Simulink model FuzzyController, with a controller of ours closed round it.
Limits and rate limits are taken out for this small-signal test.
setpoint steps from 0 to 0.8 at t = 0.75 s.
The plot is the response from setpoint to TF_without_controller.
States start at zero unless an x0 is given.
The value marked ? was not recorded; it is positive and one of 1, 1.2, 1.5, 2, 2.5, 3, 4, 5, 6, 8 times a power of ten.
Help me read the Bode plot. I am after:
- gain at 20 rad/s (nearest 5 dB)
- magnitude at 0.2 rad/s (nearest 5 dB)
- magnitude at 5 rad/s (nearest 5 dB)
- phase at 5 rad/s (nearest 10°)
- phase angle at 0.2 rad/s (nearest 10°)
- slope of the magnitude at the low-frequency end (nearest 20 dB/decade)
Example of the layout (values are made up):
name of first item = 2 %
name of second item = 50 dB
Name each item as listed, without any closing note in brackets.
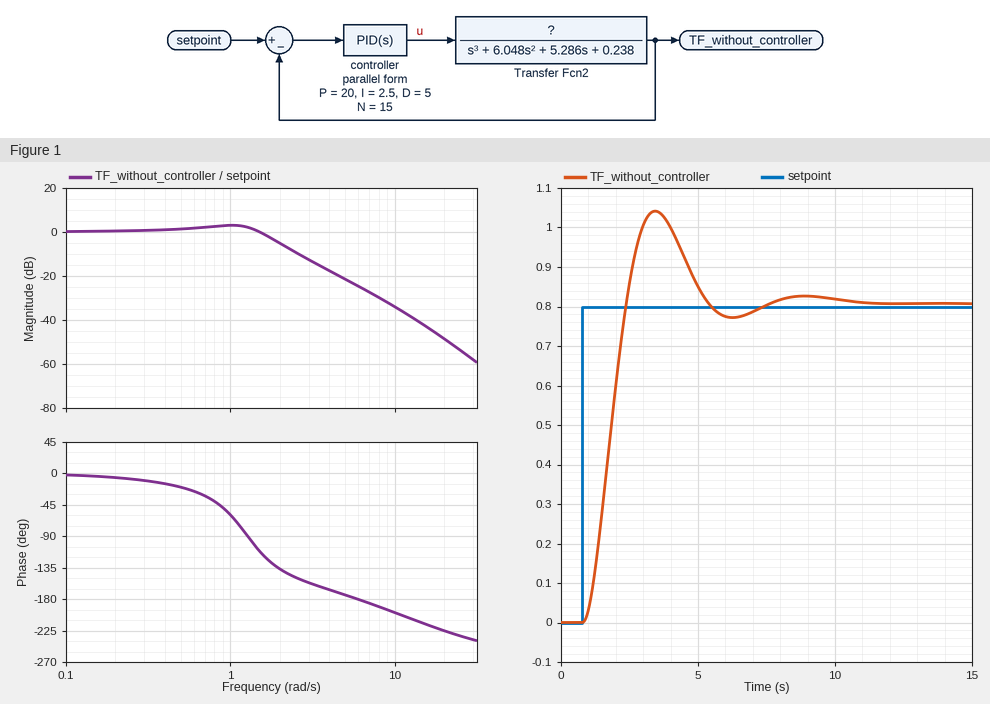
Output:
gain at 20 rad/s = -50 dB
magnitude at 0.2 rad/s = 0 dB
magnitude at 5 rad/s = -20 dB
phase at 5 rad/s = -170°
phase angle at 0.2 rad/s = -10°
slope of the magnitude at the low-frequency end = 0 dB/decade
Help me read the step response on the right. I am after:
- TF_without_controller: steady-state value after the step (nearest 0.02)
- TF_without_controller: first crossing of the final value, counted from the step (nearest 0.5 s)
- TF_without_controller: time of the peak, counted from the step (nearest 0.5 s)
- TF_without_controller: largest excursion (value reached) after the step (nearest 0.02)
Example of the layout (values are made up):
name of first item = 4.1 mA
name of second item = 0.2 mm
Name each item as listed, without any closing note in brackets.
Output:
TF_without_controller: steady-state value after the step = 0.80
TF_without_controller: first crossing of the final value, counted from the step = 1.5 s
TF_without_controller: time of the peak, counted from the step = 2.5 s
TF_without_controller: largest excursion (value reached) after the step = 1.04
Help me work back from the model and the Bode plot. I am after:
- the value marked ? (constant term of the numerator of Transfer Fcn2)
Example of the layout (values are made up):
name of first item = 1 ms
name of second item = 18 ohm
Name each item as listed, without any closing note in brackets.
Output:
the value marked ? = 0.4
